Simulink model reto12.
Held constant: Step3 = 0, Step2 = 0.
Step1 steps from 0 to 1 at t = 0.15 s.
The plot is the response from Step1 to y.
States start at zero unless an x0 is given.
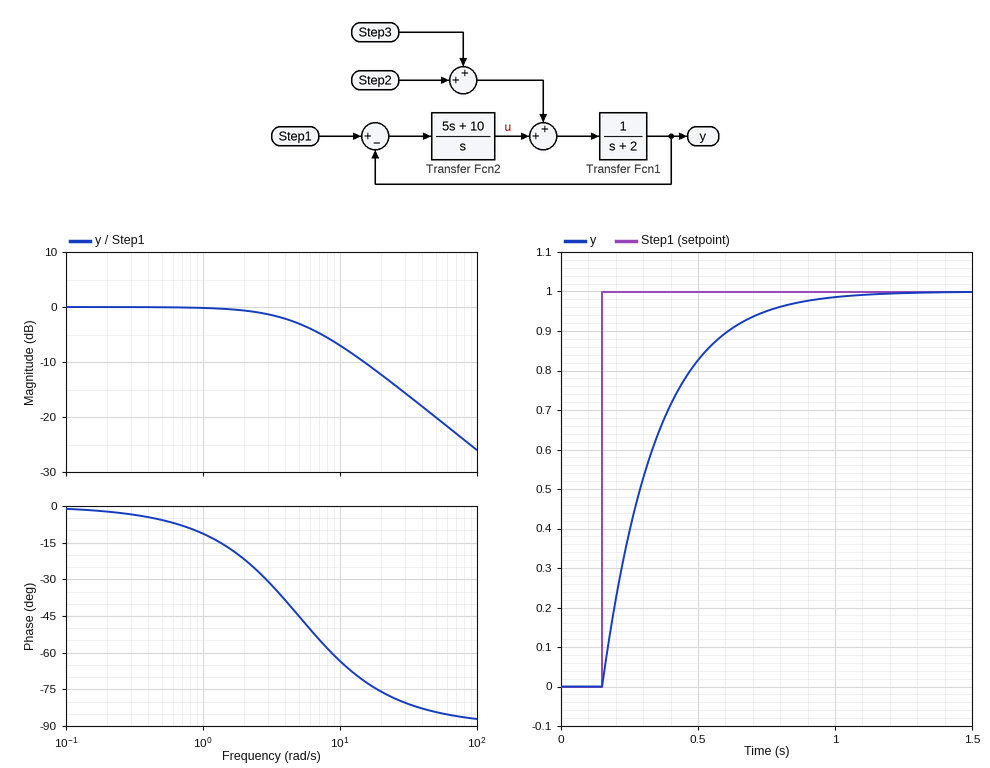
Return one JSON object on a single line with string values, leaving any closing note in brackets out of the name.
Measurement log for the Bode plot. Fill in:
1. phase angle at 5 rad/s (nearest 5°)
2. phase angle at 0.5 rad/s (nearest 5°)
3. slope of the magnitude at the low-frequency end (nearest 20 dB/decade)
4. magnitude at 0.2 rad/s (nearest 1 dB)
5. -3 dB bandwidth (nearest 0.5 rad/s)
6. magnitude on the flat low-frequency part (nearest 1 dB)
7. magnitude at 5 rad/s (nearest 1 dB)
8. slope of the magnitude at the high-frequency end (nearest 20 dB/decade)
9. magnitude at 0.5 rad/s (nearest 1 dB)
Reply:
{"phase angle at 5 rad/s": "-45°", "phase angle at 0.5 rad/s": "-5°", "slope of the magnitude at the low-frequency end": "0 dB/decade", "magnitude at 0.2 rad/s": "0 dB", "-3 dB bandwidth": "5.0 rad/s", "magnitude on the flat low-frequency part": "0 dB", "magnitude at 5 rad/s": "-3 dB", "slope of the magnitude at the high-frequency end": "-20 dB/decade", "magnitude at 0.5 rad/s": "0 dB"}
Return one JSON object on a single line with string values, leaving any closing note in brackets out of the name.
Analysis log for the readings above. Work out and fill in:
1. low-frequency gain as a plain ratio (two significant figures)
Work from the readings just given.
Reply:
{"low-frequency gain as a plain ratio": "1.0"}
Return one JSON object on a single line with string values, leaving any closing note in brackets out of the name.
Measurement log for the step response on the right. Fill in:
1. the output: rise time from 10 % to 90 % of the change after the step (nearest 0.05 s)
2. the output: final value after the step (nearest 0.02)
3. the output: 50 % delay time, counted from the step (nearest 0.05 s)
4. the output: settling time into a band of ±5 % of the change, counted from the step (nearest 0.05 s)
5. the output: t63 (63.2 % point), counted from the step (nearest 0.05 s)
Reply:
{"the output: rise time from 10 % to 90 % of the change after the step": "0.45 s", "the output: final value after the step": "1.00", "the output: 50 % delay time, counted from the step": "0.15 s", "the output: settling time into a band of ±5 % of the change, counted from the step": "0.60 s", "the output: t63 (63.2 % point), counted from the step": "0.20 s"}
